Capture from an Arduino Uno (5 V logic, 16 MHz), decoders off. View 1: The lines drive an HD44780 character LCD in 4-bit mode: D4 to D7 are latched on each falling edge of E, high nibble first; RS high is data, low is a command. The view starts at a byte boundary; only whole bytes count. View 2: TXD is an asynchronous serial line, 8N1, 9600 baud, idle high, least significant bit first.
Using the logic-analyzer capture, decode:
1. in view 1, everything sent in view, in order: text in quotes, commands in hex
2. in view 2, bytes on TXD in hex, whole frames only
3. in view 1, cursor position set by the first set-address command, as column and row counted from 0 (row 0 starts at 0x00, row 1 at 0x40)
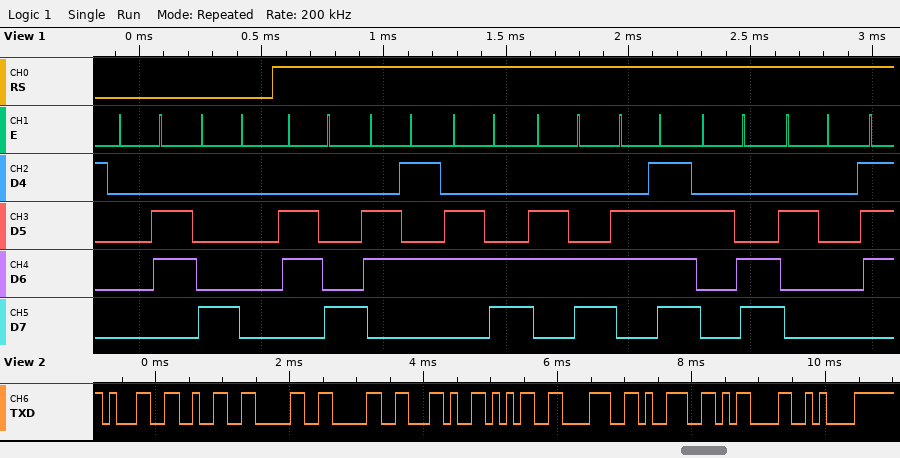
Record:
0x06 0x80 "hello, "
31 32 30 30 2C 35 38 39 0D 0A
column 0, row 0
